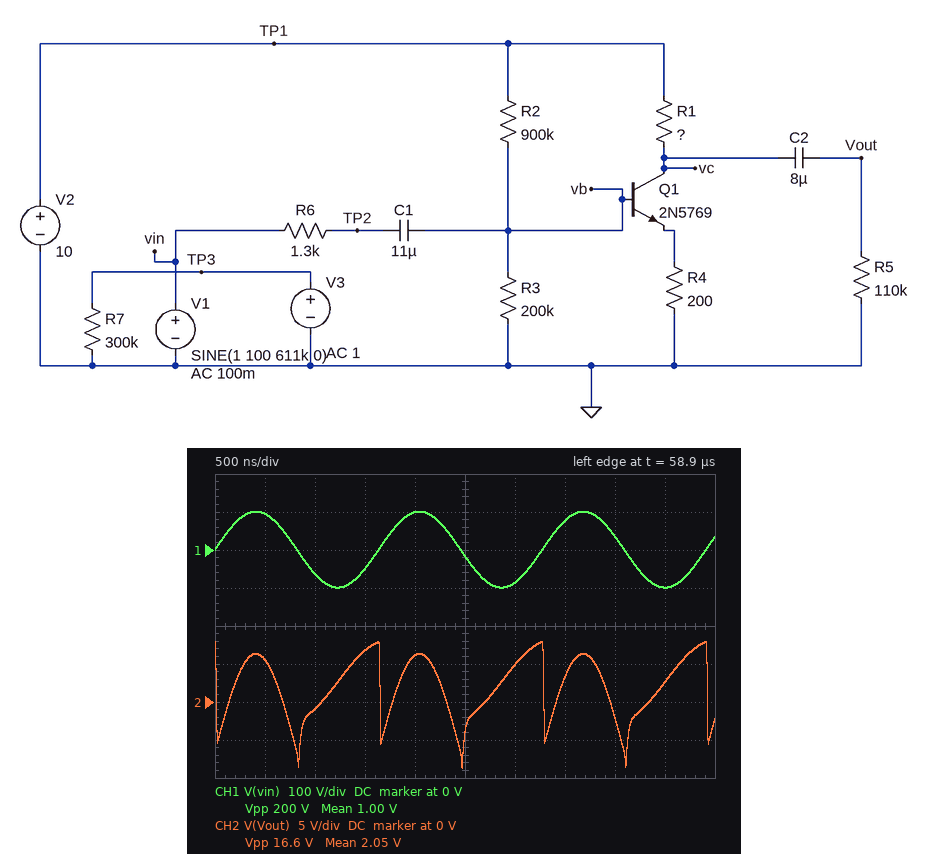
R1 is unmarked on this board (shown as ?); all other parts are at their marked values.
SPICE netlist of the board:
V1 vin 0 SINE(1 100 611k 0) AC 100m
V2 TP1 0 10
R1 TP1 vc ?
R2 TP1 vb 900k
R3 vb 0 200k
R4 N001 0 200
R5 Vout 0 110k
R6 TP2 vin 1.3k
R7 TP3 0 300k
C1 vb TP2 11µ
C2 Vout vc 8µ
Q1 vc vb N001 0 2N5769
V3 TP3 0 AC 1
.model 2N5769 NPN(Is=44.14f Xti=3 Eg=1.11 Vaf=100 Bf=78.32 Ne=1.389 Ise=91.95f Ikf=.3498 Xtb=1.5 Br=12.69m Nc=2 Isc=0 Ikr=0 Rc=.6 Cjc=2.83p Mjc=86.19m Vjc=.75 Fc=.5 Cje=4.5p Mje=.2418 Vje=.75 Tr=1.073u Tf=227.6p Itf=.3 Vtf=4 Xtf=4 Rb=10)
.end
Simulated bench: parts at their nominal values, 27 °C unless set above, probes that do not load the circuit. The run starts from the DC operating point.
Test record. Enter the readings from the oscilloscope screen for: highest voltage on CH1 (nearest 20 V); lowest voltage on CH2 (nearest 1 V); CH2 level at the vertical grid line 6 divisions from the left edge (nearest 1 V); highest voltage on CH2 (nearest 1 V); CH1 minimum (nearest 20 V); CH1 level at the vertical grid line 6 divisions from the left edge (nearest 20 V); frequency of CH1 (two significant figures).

100 V
-9 V
5 V
8 V
-100 V
-80 V
610 kHz
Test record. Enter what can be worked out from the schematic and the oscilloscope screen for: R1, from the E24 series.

6.8 kΩ
